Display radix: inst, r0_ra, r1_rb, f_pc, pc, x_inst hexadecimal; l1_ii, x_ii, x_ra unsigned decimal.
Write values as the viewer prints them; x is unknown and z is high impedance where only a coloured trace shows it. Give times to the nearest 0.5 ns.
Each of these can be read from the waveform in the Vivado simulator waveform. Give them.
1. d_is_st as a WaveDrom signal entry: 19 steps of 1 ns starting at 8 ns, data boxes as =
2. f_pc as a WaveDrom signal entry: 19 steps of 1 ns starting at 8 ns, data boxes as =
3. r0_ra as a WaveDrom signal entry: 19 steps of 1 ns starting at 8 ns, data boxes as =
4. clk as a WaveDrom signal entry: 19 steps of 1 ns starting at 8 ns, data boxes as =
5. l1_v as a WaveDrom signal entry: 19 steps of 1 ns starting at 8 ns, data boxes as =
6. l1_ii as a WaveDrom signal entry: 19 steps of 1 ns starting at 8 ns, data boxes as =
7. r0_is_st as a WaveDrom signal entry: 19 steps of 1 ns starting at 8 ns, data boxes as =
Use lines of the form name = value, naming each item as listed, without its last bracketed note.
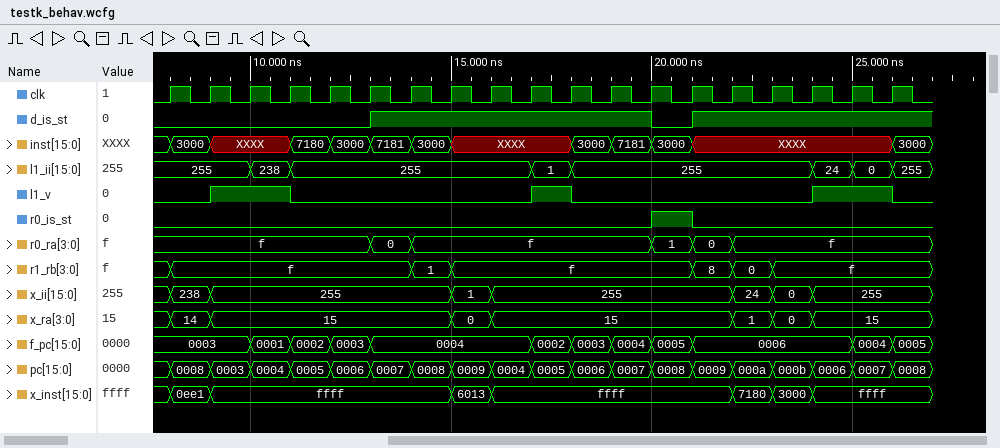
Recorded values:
d_is_st as a WaveDrom signal entry: 19 steps of 1 ns starting at 8 ns, data boxes as = = {name: 'd_is_st', wave: '0....1......01.....'}
f_pc as a WaveDrom signal entry: 19 steps of 1 ns starting at 8 ns, data boxes as = = {name: 'f_pc', wave: '=.====...=====...==', data: '0003 0001 0002 0003 0004 0002 0003 0004 0005 0006 0004 0005'}
r0_ra as a WaveDrom signal entry: 19 steps of 1 ns starting at 8 ns, data boxes as = = {name: 'r0_ra', wave: '=....==.....===....', data: 'f 0 f 1 0 f'}
clk as a WaveDrom signal entry: 19 steps of 1 ns starting at 8 ns, data boxes as = = {name: 'clk', wave: 'p..................'}
l1_v as a WaveDrom signal entry: 19 steps of 1 ns starting at 8 ns, data boxes as = = {name: 'l1_v', wave: '01.0.....10.....1.0'}
l1_ii as a WaveDrom signal entry: 19 steps of 1 ns starting at 8 ns, data boxes as = = {name: 'l1_ii', wave: '=.==.....==.....===', data: '255 238 255 1 255 24 0 255'}
r0_is_st as a WaveDrom signal entry: 19 steps of 1 ns starting at 8 ns, data boxes as = = {name: 'r0_is_st', wave: '0...........10.....'}
